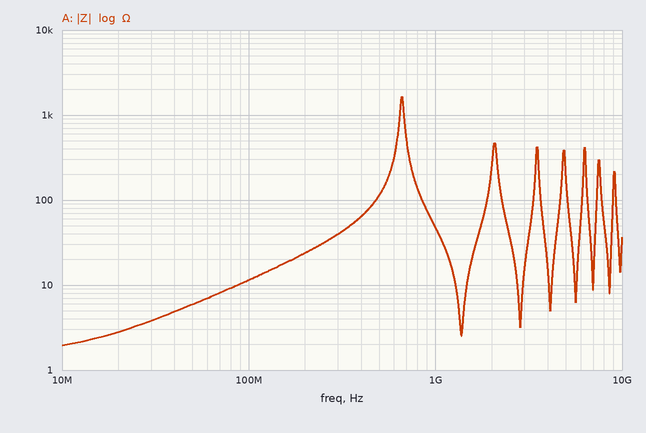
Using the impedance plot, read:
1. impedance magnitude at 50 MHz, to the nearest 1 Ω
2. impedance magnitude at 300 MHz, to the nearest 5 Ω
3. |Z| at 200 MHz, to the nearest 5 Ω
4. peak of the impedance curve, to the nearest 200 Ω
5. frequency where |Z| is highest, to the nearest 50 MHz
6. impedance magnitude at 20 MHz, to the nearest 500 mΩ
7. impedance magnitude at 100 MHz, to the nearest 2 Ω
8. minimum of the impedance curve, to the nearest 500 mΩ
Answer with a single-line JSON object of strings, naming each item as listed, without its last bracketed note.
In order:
{"impedance magnitude at 50 MHz, to the nearest 1 Ω": "6 Ω", "impedance magnitude at 300 MHz, to the nearest 5 Ω": "40 Ω", "|Z| at 200 MHz, to the nearest 5 Ω": "25 Ω", "peak of the impedance curve, to the nearest 200 Ω": "1.6 kΩ", "frequency where |Z| is highest, to the nearest 50 MHz": "650 MHz", "impedance magnitude at 20 MHz, to the nearest 500 mΩ": "3.0 Ω", "impedance magnitude at 100 MHz, to the nearest 2 Ω": "12 Ω", "minimum of the impedance curve, to the nearest 500 mΩ": "2.0 Ω"}
